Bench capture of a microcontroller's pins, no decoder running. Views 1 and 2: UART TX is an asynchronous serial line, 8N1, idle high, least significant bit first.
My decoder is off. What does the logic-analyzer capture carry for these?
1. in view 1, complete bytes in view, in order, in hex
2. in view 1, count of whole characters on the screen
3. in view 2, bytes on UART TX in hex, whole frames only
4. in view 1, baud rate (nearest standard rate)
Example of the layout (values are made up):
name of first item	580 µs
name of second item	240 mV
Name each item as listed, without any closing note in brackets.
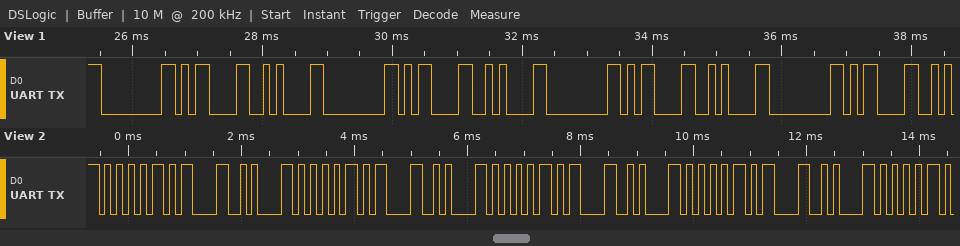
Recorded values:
in view 1, complete bytes in view, in order, in hex	00 0D 0A 00 0D 0A 00 0D 0A 00 0D
in view 1, count of whole characters on the screen	11
in view 2, bytes on UART TX in hex, whole frames only	0x55 0x0D 0x0A 0x55 0x0D 0x0A 0x55 0x0D 0x0A 0x55 0x0D 0x0A 0x55
in view 1, baud rate	9600 baud
